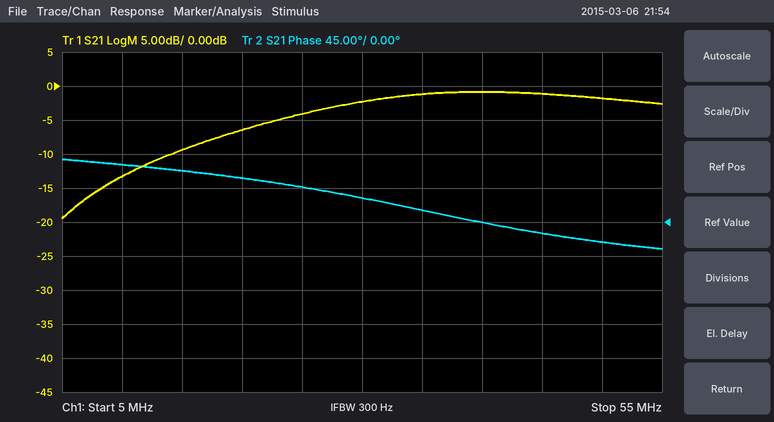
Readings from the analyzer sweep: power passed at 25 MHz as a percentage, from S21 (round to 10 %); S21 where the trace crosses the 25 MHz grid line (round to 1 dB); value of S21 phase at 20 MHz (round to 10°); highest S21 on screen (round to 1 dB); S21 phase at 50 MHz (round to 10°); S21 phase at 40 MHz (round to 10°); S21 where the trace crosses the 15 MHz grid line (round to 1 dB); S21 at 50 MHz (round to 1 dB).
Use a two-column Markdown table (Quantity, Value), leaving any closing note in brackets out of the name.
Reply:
| Quantity | Value |
|---|---|
| power passed at 25 MHz as a percentage, from S21 | 40 % |
| S21 where the trace crosses the 25 MHz grid line | -4 dB |
| value of S21 phase at 20 MHz | 60° |
| highest S21 on screen | -1 dB |
| S21 phase at 50 MHz | -30° |
| S21 phase at 40 MHz | 0° |
| S21 where the trace crosses the 15 MHz grid line | -9 dB |
| S21 at 50 MHz | -2 dB |
